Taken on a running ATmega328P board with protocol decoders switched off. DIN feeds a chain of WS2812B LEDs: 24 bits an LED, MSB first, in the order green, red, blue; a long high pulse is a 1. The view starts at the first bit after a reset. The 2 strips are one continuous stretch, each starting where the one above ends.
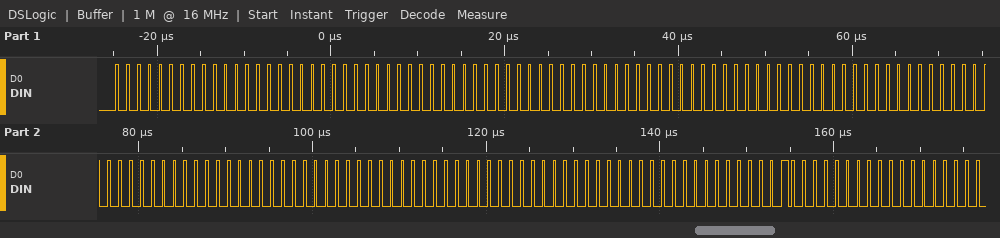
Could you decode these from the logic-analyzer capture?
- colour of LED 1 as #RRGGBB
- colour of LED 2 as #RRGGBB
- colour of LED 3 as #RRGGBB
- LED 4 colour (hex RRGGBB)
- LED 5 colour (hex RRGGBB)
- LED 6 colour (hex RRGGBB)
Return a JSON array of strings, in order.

["#000000", "#000000", "#000000", "#000000", "#000000", "#000001"]
